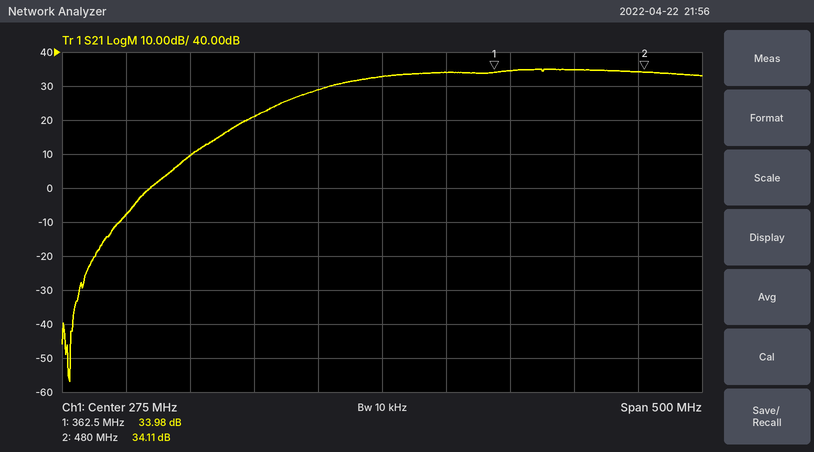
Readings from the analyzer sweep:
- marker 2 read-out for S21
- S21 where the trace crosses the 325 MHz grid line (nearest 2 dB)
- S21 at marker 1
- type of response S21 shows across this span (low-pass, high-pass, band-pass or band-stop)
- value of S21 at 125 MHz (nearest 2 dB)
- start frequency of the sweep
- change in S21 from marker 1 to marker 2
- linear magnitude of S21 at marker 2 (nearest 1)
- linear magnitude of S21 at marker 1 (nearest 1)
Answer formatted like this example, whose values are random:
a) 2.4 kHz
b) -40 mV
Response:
a) 34.11 dB
b) 34 dB
c) 33.98 dB
d) high-pass
e) 10 dB
f) 25 MHz
g) 0.13 dB
h) 51
i) 50
